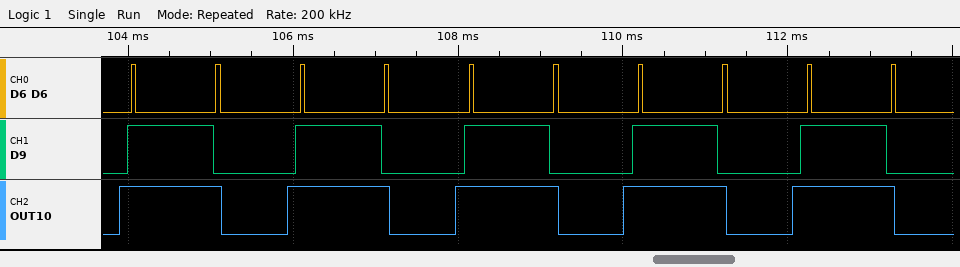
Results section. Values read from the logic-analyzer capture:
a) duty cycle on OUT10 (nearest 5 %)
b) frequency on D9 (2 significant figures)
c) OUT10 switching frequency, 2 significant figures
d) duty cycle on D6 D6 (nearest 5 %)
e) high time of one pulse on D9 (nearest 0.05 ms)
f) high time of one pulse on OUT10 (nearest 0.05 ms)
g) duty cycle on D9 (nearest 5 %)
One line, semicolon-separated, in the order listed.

60 %; 490 Hz; 490 Hz; 5 %; 1.05 ms; 1.25 ms; 50 %
